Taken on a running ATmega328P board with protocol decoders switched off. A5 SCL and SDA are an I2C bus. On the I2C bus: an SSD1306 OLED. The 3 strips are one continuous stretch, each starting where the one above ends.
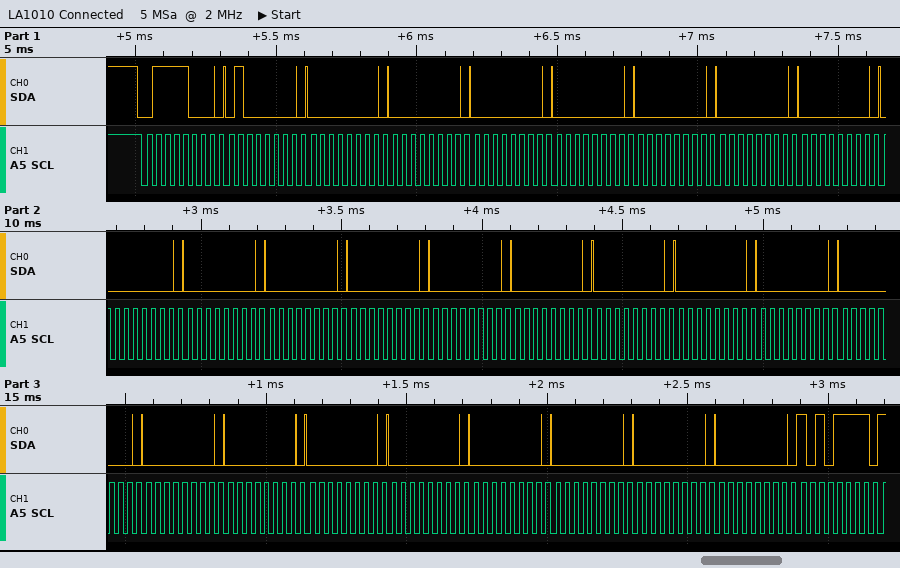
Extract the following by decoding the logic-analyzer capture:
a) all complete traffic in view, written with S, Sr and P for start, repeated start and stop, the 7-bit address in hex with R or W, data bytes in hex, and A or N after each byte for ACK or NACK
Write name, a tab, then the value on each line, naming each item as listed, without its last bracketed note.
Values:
all complete traffic in view, written with S, Sr and P for start, repeated start and stop, the 7-bit address in hex with R or W, data bytes in hex, and A or N after each byte for ACK or NACK	S 3CW A 40 A 00 A 00 A 00 A 00 A 00 A 00 A 00 A 00 A 00 A 00 A 00 A 00 A 00 A 00 A 00 A 00 A 00 A 00 A 00 A 00 A 00 A 00 A 00 A 00 A 00 A AF A
